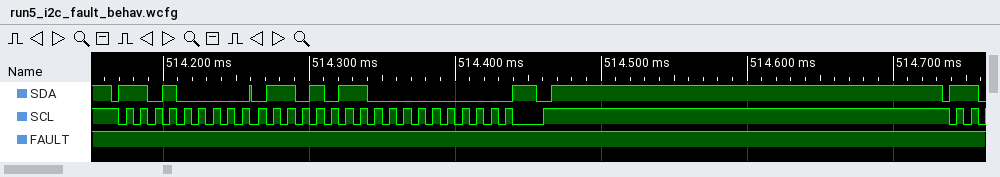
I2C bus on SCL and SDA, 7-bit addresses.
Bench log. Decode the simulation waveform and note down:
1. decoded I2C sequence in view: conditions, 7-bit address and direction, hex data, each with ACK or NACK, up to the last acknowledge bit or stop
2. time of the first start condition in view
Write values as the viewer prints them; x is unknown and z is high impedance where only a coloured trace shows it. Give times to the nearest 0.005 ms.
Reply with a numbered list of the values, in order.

1. start, address 68 write ACK, 6B ACK, 00 ACK, stop
2. 514.165 ms
